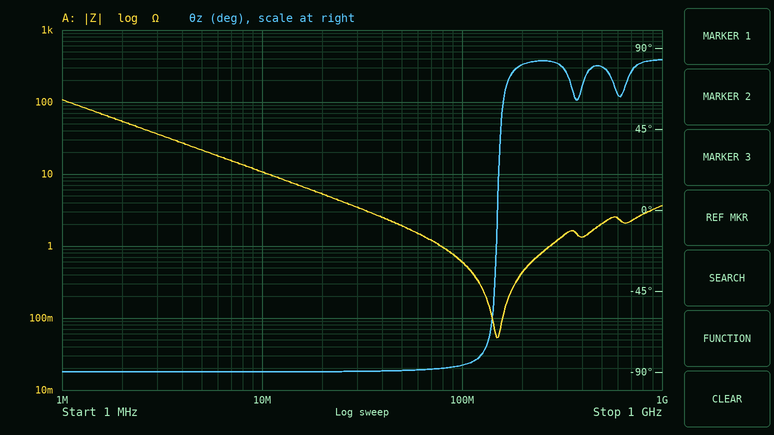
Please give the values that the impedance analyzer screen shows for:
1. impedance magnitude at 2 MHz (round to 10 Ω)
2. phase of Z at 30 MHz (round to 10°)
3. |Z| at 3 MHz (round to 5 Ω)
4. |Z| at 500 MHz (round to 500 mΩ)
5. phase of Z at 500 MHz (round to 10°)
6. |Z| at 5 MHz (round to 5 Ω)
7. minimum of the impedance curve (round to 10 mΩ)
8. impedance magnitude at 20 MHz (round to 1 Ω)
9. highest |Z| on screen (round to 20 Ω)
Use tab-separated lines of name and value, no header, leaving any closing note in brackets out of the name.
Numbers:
impedance magnitude at 2 MHz	50 Ω
phase of Z at 30 MHz	-90°
|Z| at 3 MHz	35 Ω
|Z| at 500 MHz	2.0 Ω
phase of Z at 500 MHz	80°
|Z| at 5 MHz	20 Ω
minimum of the impedance curve	50 mΩ
impedance magnitude at 20 MHz	5 Ω
highest |Z| on screen	100 Ω
